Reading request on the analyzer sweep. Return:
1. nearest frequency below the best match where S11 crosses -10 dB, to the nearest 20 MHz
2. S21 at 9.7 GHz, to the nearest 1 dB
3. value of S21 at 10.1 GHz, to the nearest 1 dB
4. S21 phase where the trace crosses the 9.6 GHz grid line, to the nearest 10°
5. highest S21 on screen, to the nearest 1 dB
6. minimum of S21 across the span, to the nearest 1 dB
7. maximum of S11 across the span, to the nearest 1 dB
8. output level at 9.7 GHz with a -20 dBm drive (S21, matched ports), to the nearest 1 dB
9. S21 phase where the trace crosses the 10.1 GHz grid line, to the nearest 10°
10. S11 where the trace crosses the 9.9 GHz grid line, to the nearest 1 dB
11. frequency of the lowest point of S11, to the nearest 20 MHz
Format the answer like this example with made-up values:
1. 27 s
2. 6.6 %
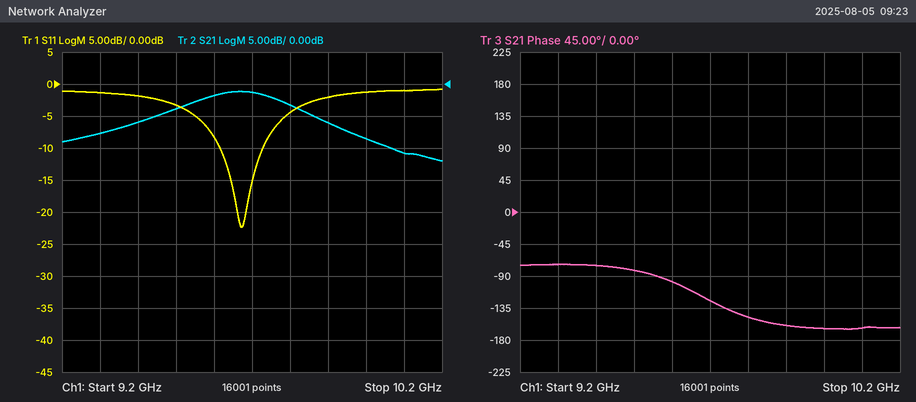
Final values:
1. 9.62 GHz
2. -1 dB
3. -11 dB
4. -100°
5. -1 dB
6. -12 dB
7. -1 dB
8. -21 dBm
9. -160°
10. -2 dB
11. 9.68 GHz
